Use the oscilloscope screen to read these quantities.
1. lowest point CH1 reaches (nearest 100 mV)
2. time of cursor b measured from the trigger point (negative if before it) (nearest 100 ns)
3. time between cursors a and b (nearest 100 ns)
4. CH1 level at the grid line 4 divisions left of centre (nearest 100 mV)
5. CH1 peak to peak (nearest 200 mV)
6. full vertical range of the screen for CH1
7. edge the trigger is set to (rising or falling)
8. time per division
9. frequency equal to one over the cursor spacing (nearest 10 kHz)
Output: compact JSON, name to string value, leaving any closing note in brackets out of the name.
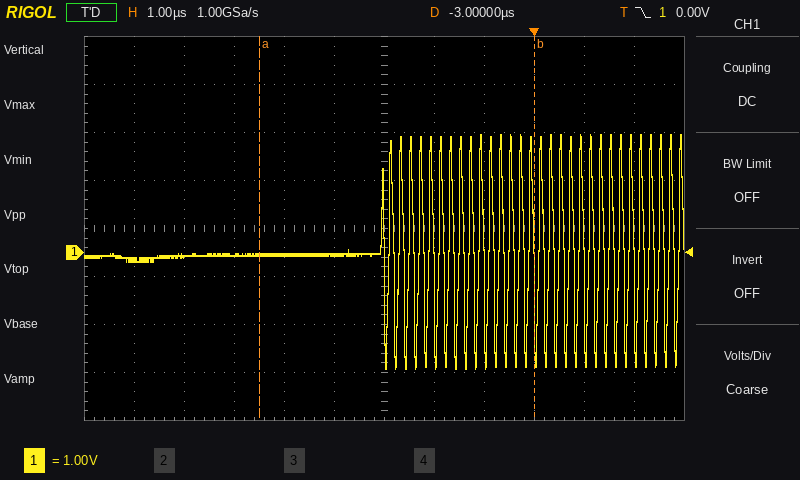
{"lowest point CH1 reaches": "-2.4 V", "time of cursor b measured from the trigger point (negative if before it)": "0.0 µs", "time between cursors a and b": "5.5 µs", "CH1 level at the grid line 4 divisions left of centre": "-100 mV", "CH1 peak to peak": "4.8 V", "full vertical range of the screen for CH1": "8 V", "edge the trigger is set to": "falling", "time per division": "1 µs", "frequency equal to one over the cursor spacing": "180 kHz"}
